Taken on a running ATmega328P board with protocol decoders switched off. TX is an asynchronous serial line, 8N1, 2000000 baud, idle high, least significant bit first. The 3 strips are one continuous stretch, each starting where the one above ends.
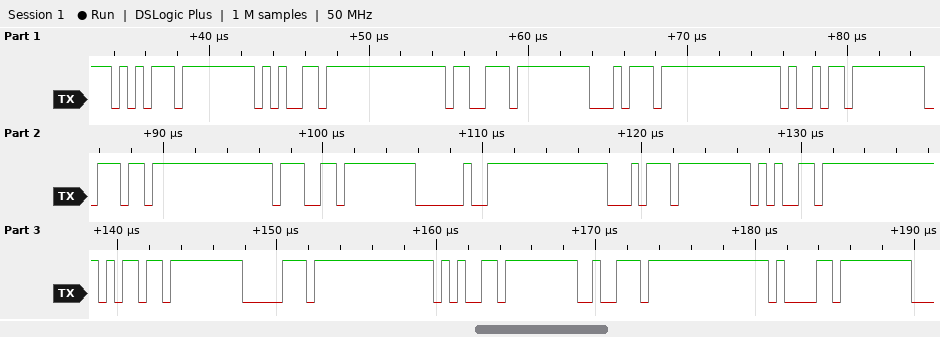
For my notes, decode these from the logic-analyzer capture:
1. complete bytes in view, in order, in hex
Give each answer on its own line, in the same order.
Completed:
0x75 0x65 0x73 0x74 0x69 0x6E 0x67 0x20 0x74 0x65 0x6D 0x70 0x65 0x72 0x61
